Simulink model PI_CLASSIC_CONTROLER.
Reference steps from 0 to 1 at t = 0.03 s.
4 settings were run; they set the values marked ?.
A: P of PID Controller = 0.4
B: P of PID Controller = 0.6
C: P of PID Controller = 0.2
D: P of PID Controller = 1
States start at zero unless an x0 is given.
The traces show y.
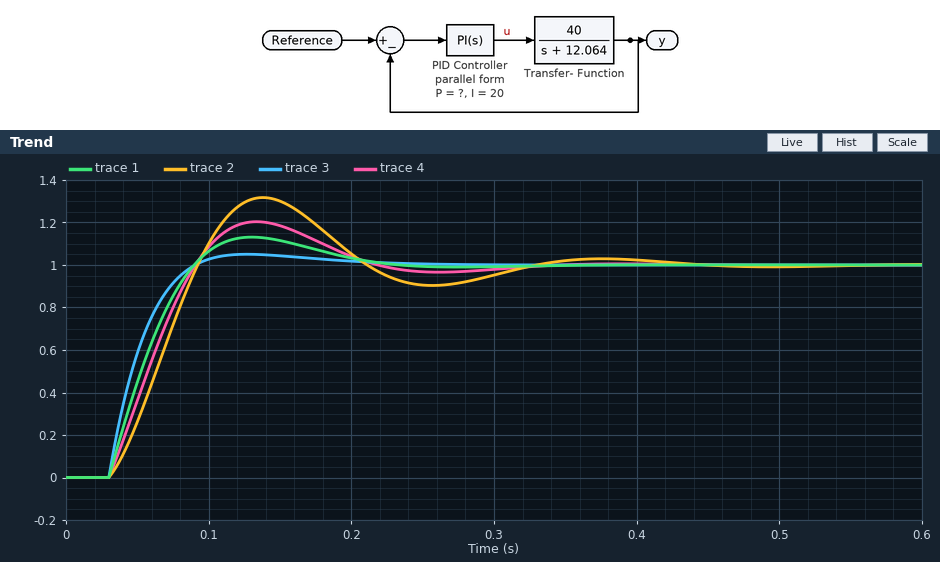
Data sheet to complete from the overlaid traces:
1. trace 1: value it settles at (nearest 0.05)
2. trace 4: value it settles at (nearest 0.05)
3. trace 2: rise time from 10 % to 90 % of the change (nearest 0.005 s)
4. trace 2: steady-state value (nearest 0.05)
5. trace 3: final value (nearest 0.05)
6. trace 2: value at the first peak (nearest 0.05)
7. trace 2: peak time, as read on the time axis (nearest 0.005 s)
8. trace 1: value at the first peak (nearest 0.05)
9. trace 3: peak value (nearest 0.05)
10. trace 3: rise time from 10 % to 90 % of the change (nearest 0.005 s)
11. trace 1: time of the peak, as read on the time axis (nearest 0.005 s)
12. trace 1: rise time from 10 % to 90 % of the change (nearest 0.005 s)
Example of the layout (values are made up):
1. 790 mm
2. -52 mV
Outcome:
1. 1.00
2. 1.00
3. 0.045 s
4. 1.00
5. 1.00
6. 1.30
7. 0.140 s
8. 1.15
9. 1.05
10. 0.040 s
11. 0.130 s
12. 0.045 s
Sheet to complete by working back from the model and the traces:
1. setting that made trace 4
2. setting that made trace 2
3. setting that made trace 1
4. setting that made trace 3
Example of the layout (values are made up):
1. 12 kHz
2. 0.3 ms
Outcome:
1. A
2. C
3. B
4. D
